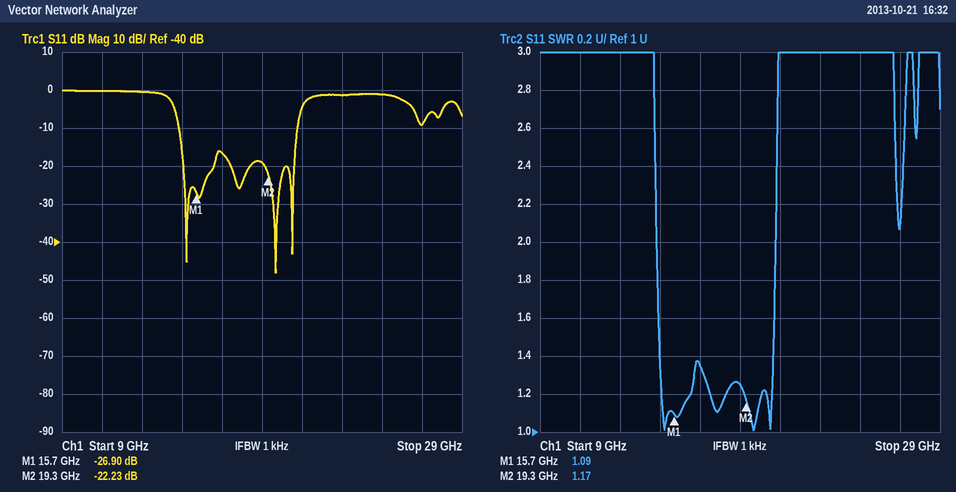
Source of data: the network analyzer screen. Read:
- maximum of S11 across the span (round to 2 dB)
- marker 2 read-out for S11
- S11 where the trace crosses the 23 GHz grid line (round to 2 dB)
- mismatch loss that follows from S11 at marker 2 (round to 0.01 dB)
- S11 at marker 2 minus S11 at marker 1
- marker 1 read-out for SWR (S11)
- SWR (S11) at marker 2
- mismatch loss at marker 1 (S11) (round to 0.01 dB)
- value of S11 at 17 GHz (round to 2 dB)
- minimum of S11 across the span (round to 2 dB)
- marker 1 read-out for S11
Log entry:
0 dB
-22.23 dB
-2 dB
0.03 dB
4.67 dB
1.09
1.17
0.01 dB
-16 dB
-48 dB
-26.90 dB
